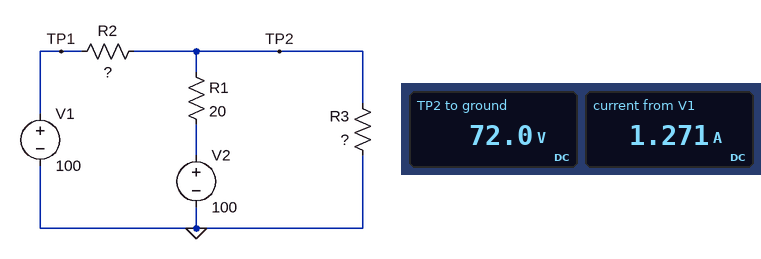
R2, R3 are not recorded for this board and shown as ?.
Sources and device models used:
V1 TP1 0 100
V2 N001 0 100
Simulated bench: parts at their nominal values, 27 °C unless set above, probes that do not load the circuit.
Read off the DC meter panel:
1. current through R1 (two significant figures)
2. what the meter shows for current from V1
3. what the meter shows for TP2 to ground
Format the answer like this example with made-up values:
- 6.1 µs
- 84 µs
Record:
- 1.4 A
- 1.271 A
- 72.0 V
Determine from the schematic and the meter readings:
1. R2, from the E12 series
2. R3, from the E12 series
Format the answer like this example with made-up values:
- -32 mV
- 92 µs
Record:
- 22 Ω
- 27 Ω
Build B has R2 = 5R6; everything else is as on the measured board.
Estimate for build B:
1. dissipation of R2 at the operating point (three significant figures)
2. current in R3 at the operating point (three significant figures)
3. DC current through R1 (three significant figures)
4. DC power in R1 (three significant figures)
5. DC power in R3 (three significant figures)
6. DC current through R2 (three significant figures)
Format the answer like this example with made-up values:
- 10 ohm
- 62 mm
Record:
- 34.7 W
- 3.19 A
- 697 mA
- 9.72 W
- 274 W
- 2.49 A
